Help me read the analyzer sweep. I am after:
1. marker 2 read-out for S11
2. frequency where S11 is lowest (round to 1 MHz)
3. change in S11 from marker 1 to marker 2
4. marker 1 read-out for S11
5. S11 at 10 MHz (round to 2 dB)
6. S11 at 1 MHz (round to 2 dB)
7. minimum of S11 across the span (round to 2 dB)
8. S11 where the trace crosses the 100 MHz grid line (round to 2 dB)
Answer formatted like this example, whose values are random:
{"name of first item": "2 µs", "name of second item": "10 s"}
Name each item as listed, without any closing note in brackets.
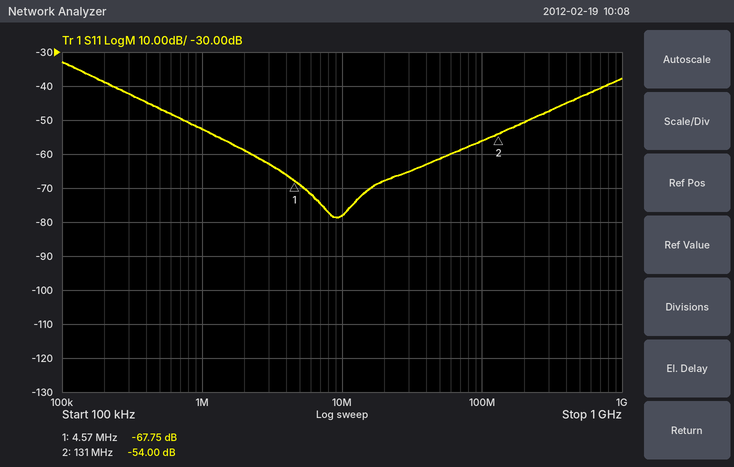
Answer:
{"marker 2 read-out for S11": "-54.00 dB", "frequency where S11 is lowest": "9 MHz", "change in S11 from marker 1 to marker 2": "13.75 dB", "marker 1 read-out for S11": "-67.75 dB", "S11 at 10 MHz": "-78 dB", "S11 at 1 MHz": "-52 dB", "minimum of S11 across the span": "-78 dB", "S11 where the trace crosses the 100 MHz grid line": "-56 dB"}
